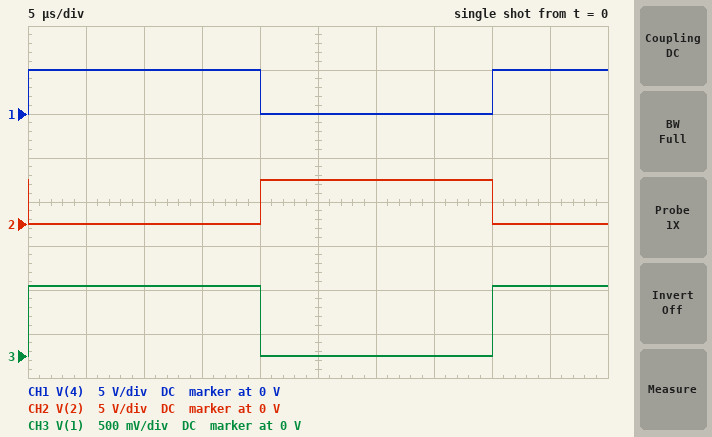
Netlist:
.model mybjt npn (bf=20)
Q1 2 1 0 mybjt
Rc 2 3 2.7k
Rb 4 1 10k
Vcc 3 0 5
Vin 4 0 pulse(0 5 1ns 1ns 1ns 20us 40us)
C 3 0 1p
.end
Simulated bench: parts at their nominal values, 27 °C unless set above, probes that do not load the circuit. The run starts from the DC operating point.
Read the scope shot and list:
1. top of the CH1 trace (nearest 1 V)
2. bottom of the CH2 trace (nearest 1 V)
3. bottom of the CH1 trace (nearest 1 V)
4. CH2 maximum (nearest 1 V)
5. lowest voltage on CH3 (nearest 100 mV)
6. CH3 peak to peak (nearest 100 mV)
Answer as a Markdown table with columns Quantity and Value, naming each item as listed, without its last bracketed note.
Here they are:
| Quantity | Value |
|---|---|
| top of the CH1 trace | 5 V |
| bottom of the CH2 trace | 0 V |
| bottom of the CH1 trace | 0 V |
| CH2 maximum | 5 V |
| lowest voltage on CH3 | 0 V |
| CH3 peak to peak | 800 mV |
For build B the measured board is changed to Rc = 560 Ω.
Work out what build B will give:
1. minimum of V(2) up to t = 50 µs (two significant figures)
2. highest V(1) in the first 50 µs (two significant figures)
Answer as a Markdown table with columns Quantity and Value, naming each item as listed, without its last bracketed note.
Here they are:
| Quantity | Value |
|---|---|
| minimum of V(2) up to t = 50 µs | 330 mV |
| highest V(1) in the first 50 µs | 830 mV |
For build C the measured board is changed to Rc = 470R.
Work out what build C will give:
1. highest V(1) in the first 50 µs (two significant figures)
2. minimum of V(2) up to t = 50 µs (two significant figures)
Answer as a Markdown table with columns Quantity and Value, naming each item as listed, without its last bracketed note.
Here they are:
| Quantity | Value |
|---|---|
| highest V(1) in the first 50 µs | 830 mV |
| minimum of V(2) up to t = 50 µs | 1.1 V |
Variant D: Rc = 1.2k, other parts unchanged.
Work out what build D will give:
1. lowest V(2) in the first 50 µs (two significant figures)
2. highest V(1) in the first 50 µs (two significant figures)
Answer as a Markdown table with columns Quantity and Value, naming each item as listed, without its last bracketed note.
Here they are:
| Quantity | Value |
|---|---|
| lowest V(2) in the first 50 µs | 81 mV |
| highest V(1) in the first 50 µs | 810 mV |
